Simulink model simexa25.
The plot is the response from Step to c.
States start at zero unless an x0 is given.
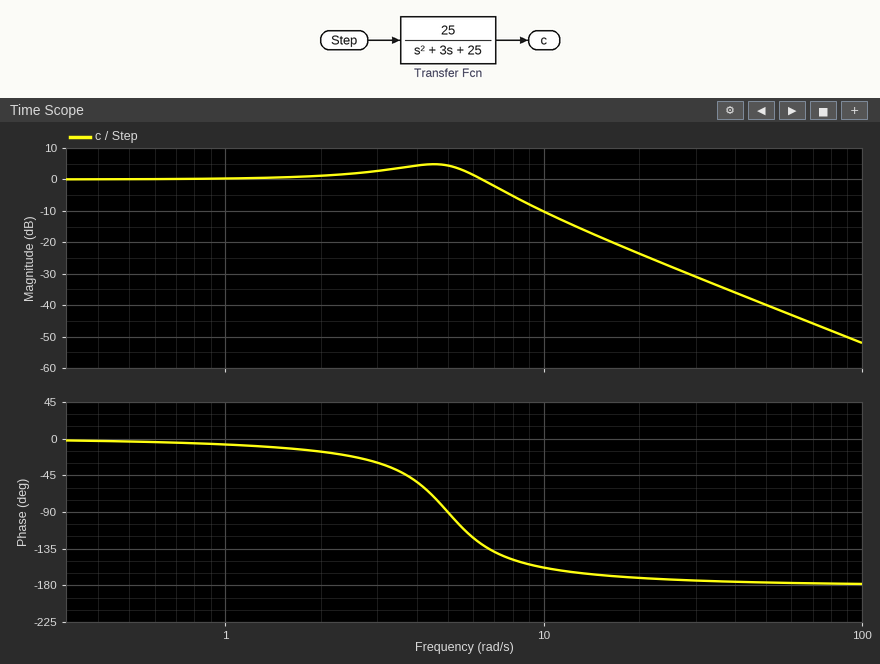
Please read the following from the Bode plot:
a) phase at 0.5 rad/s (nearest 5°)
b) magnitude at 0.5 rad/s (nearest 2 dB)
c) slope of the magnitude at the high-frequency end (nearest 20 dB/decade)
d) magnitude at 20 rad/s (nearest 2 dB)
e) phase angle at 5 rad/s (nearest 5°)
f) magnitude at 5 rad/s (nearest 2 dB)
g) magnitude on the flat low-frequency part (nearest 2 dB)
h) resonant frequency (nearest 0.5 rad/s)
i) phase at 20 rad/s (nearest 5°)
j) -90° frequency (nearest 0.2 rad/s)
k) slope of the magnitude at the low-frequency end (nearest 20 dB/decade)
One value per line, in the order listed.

-5°
0 dB
-40 dB/decade
-24 dB
-90°
4 dB
0 dB
4.5 rad/s
-170°
5.0 rad/s
0 dB/decade
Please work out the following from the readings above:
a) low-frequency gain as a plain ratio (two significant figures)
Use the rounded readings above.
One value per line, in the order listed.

1.0
